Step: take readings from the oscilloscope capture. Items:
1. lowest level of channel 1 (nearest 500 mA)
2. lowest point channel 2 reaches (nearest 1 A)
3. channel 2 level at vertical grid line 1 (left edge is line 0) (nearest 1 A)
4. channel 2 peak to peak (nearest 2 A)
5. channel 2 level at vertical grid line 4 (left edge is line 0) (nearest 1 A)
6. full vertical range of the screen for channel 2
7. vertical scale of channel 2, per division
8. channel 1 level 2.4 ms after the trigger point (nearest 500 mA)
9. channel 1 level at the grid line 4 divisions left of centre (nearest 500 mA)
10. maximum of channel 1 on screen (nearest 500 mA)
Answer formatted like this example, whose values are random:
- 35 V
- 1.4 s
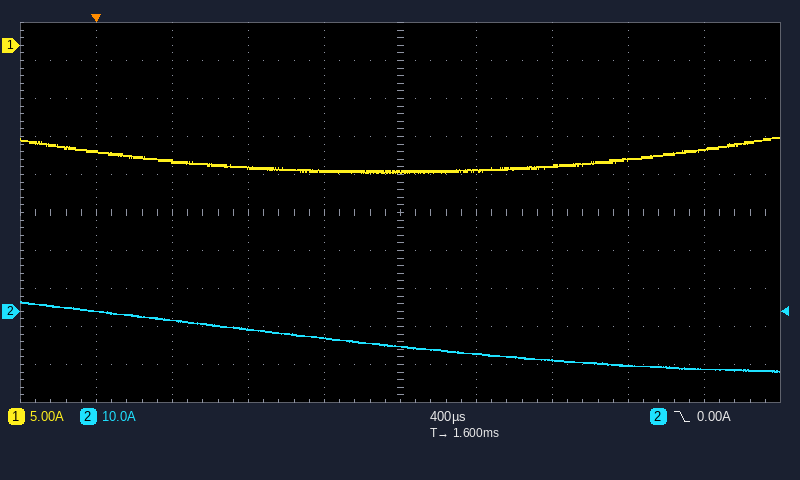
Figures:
- -17.0 A
- -16 A
- 0 A
- 18 A
- -7 A
- 100 A
- 10 A
- -16.0 A
- -14.0 A
- -12.0 A
